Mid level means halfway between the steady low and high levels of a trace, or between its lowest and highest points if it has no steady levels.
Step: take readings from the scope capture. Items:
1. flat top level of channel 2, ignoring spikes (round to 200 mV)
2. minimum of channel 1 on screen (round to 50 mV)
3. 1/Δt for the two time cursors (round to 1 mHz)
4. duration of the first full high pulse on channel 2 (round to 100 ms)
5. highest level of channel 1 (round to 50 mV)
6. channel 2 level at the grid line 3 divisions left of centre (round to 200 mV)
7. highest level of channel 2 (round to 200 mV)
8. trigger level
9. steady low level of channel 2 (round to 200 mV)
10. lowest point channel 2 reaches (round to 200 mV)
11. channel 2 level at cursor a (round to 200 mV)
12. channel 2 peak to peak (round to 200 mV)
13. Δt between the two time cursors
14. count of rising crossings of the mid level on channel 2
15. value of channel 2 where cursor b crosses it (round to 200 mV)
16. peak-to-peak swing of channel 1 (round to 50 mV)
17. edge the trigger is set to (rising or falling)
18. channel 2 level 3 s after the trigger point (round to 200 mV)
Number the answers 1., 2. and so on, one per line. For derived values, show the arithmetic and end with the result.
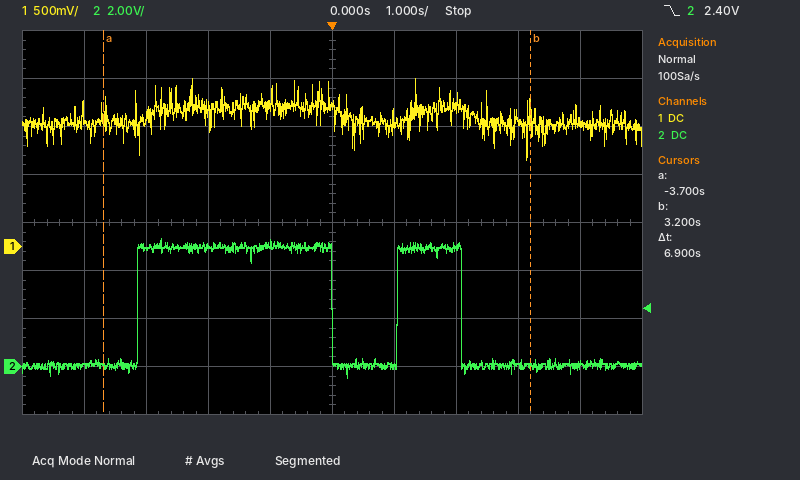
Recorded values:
1. 5.0 V
2. 900 mV
3. 1 / 6.9 s ≈ 145 mHz
4. 3.1 s
5. 1.75 V
6. 5.0 V
7. 5.4 V
8. 2.40 V
9. 0.0 V
10. -400 mV
11. 0.0 V
12. 5.4 V − (-400 mV) = 5.8 V
13. 6.9 s
14. 2
15. 0.0 V
16. 1.75 V − (900 mV) = 850 mV
17. falling
18. 0.0 V
